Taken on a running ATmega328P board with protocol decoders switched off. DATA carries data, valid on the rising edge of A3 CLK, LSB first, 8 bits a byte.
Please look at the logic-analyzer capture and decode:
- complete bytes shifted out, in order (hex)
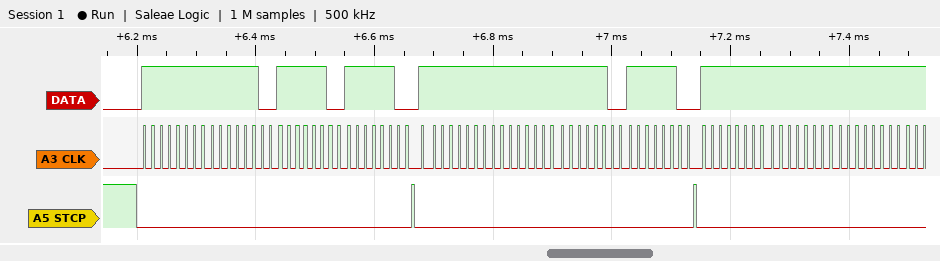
FF 3F 3F 3F FF FF 3F 3F FF FF FF
